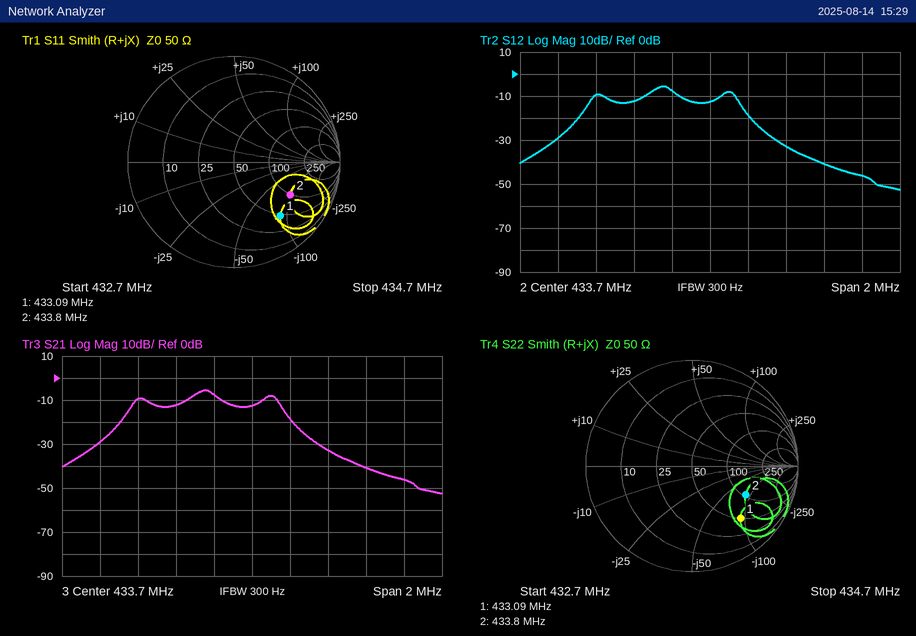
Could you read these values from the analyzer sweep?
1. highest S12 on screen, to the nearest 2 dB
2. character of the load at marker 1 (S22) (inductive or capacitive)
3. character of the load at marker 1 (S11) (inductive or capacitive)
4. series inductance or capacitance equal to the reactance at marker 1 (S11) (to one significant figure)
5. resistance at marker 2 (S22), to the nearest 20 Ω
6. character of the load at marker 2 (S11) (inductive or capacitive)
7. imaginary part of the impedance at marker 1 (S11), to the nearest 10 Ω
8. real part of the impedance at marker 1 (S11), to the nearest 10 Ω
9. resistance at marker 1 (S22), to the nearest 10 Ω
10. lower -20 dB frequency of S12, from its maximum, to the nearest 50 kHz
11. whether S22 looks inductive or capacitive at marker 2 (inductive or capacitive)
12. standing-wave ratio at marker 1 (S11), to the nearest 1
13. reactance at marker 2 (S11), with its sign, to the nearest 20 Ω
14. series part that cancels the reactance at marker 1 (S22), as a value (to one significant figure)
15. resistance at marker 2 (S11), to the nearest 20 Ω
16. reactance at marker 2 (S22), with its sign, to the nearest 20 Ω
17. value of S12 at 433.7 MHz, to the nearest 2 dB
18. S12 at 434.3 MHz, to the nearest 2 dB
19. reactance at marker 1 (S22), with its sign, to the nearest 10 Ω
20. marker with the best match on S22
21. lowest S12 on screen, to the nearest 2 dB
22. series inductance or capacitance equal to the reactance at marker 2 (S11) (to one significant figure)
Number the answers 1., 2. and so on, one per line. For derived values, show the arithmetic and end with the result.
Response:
1. -6 dB
2. capacitive
3. capacitive
4. C = 1/(2π × 433.09 MHz × 90 Ω) ≈ 4 pF
5. 100 Ω
6. capacitive
7. -90 Ω
8. 50 Ω
9. 50 Ω
10. 432.95 MHz
11. capacitive
12. 5
13. -100 Ω
14. L = 90 Ω/(2π × 433.09 MHz) ≈ 33.1 nH, so 30 nH to one significant figure
15. 100 Ω
16. -80 Ω
17. -12 dB
18. -40 dB
19. -90 Ω
20. marker 2
21. -52 dB
22. C = 1/(2π × 433.8 MHz × 100 Ω) ≈ 4 pF
